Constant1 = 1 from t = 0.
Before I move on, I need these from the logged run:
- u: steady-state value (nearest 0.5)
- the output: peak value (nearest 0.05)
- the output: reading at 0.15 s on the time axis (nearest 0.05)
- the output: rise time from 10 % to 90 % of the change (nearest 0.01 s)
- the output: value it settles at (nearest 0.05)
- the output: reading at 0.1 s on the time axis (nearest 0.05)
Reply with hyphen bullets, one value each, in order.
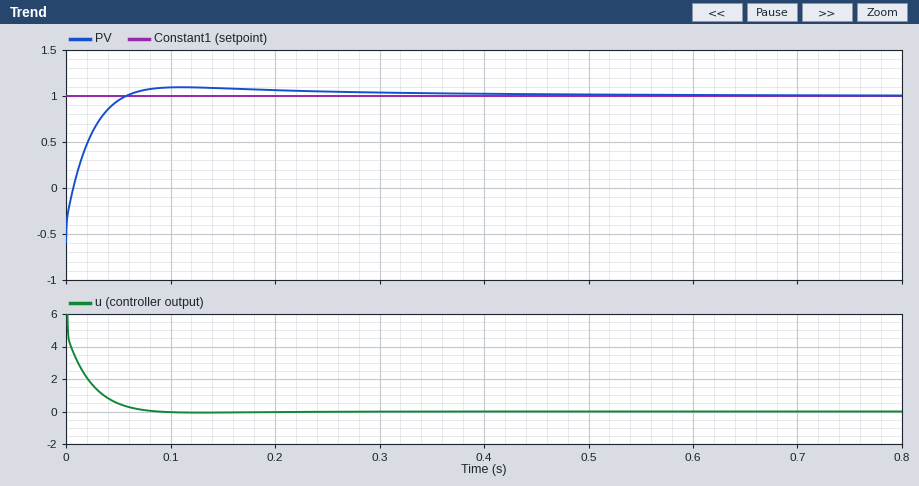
- 0.0
- 1.10
- 1.10
- 0.04 s
- 1.00
- 1.10
